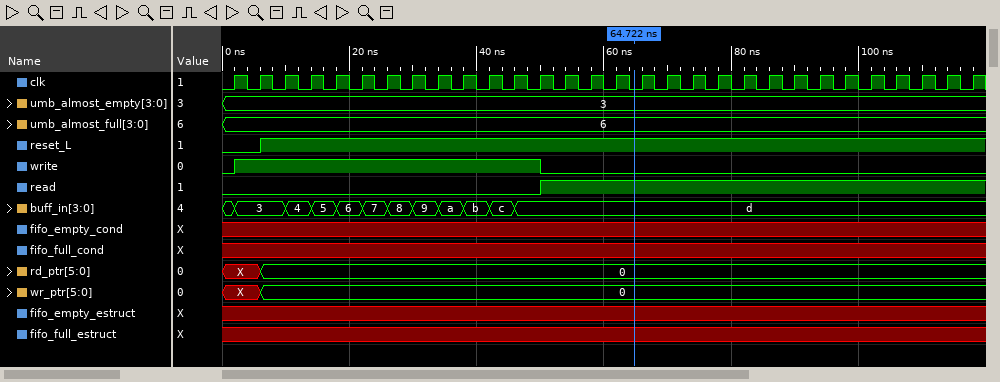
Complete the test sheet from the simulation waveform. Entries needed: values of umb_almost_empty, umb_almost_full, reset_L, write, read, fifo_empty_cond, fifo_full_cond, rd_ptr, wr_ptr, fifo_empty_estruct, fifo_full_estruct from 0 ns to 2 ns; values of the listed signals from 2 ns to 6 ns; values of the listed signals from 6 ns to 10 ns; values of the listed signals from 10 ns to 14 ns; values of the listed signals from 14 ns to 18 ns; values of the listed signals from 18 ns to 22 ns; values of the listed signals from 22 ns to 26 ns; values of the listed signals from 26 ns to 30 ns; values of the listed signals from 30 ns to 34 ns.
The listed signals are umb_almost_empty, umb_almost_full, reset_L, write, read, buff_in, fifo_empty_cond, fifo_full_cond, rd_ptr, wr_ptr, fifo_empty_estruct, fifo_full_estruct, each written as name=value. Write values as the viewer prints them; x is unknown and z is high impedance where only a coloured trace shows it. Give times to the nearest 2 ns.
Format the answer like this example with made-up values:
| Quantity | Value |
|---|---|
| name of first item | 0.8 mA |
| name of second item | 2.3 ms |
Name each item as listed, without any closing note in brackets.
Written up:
| Quantity | Value |
|---|---|
| values of umb_almost_empty, umb_almost_full, reset_L, write, read, fifo_empty_cond, fifo_full_cond, rd_ptr, wr_ptr, fifo_empty_estruct, fifo_full_estruct from 0 ns to 2 ns | umb_almost_empty=3, umb_almost_full=6, reset_L=0, write=0, read=0, fifo_empty_cond=x, fifo_full_cond=x, rd_ptr=X, wr_ptr=X, fifo_empty_estruct=x, fifo_full_estruct=x |
| values of the listed signals from 2 ns to 6 ns | umb_almost_empty=3, umb_almost_full=6, reset_L=0, write=1, read=0, buff_in=3, fifo_empty_cond=x, fifo_full_cond=x, rd_ptr=X, wr_ptr=X, fifo_empty_estruct=x, fifo_full_estruct=x |
| values of the listed signals from 6 ns to 10 ns | umb_almost_empty=3, umb_almost_full=6, reset_L=1, write=1, read=0, buff_in=3, fifo_empty_cond=x, fifo_full_cond=x, rd_ptr=0, wr_ptr=0, fifo_empty_estruct=x, fifo_full_estruct=x |
| values of the listed signals from 10 ns to 14 ns | umb_almost_empty=3, umb_almost_full=6, reset_L=1, write=1, read=0, buff_in=4, fifo_empty_cond=x, fifo_full_cond=x, rd_ptr=0, wr_ptr=0, fifo_empty_estruct=x, fifo_full_estruct=x |
| values of the listed signals from 14 ns to 18 ns | umb_almost_empty=3, umb_almost_full=6, reset_L=1, write=1, read=0, buff_in=5, fifo_empty_cond=x, fifo_full_cond=x, rd_ptr=0, wr_ptr=0, fifo_empty_estruct=x, fifo_full_estruct=x |
| values of the listed signals from 18 ns to 22 ns | umb_almost_empty=3, umb_almost_full=6, reset_L=1, write=1, read=0, buff_in=6, fifo_empty_cond=x, fifo_full_cond=x, rd_ptr=0, wr_ptr=0, fifo_empty_estruct=x, fifo_full_estruct=x |
| values of the listed signals from 22 ns to 26 ns | umb_almost_empty=3, umb_almost_full=6, reset_L=1, write=1, read=0, buff_in=7, fifo_empty_cond=x, fifo_full_cond=x, rd_ptr=0, wr_ptr=0, fifo_empty_estruct=x, fifo_full_estruct=x |
| values of the listed signals from 26 ns to 30 ns | umb_almost_empty=3, umb_almost_full=6, reset_L=1, write=1, read=0, buff_in=8, fifo_empty_cond=x, fifo_full_cond=x, rd_ptr=0, wr_ptr=0, fifo_empty_estruct=x, fifo_full_estruct=x |
| values of the listed signals from 30 ns to 34 ns | umb_almost_empty=3, umb_almost_full=6, reset_L=1, write=1, read=0, buff_in=9, fifo_empty_cond=x, fifo_full_cond=x, rd_ptr=0, wr_ptr=0, fifo_empty_estruct=x, fifo_full_estruct=x |
